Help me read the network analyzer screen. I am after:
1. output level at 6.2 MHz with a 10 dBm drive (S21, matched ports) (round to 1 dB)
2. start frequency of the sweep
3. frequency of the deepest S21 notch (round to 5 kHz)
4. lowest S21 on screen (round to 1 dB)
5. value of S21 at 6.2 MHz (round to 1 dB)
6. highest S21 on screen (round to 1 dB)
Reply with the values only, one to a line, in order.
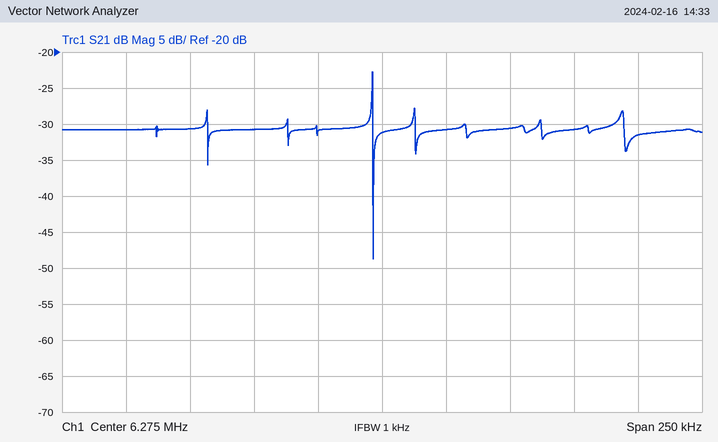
-21 dBm
6.15 MHz
6.270 MHz
-49 dB
-31 dB
-23 dB
